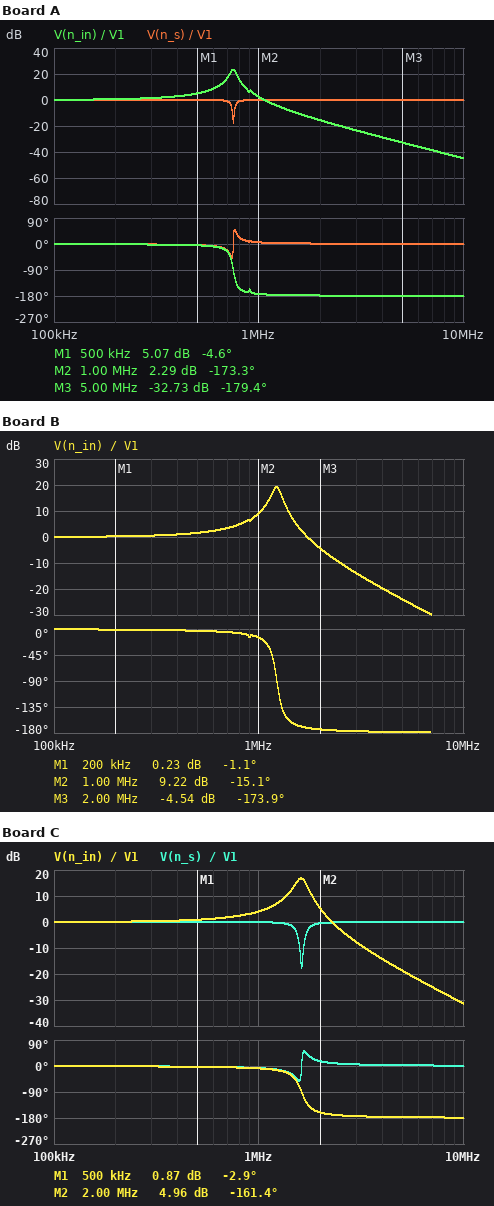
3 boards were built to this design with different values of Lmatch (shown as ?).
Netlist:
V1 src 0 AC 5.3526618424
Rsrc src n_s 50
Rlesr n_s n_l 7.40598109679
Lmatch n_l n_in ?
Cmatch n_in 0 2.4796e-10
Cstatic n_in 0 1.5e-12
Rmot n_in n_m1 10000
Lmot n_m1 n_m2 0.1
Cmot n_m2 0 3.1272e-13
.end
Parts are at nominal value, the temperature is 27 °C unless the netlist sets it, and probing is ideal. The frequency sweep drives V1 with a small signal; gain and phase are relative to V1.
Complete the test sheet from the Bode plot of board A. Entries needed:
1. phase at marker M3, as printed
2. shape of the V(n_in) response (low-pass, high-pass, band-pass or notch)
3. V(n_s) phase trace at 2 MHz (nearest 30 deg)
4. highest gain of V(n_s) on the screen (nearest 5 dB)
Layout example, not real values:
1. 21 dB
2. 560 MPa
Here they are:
1. -179.4 deg
2. low-pass
3. 0 deg
4. 0 dB
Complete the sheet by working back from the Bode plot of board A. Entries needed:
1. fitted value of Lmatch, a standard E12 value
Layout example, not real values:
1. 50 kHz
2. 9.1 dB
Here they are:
1. 180 µH
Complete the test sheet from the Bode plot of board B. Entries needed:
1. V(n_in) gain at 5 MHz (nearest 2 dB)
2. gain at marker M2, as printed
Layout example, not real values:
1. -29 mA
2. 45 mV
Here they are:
1. -24 dB
2. 9.22 dB
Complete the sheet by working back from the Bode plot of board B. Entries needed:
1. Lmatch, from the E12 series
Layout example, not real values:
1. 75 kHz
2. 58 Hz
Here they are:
1. 68 µH
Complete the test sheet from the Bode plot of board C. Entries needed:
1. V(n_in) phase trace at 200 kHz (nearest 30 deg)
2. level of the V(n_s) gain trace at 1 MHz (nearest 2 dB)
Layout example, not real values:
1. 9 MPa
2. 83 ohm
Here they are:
1. 0 deg
2. 0 dB
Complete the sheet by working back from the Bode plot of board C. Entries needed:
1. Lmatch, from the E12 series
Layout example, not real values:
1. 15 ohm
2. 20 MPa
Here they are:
1. 39 µH
